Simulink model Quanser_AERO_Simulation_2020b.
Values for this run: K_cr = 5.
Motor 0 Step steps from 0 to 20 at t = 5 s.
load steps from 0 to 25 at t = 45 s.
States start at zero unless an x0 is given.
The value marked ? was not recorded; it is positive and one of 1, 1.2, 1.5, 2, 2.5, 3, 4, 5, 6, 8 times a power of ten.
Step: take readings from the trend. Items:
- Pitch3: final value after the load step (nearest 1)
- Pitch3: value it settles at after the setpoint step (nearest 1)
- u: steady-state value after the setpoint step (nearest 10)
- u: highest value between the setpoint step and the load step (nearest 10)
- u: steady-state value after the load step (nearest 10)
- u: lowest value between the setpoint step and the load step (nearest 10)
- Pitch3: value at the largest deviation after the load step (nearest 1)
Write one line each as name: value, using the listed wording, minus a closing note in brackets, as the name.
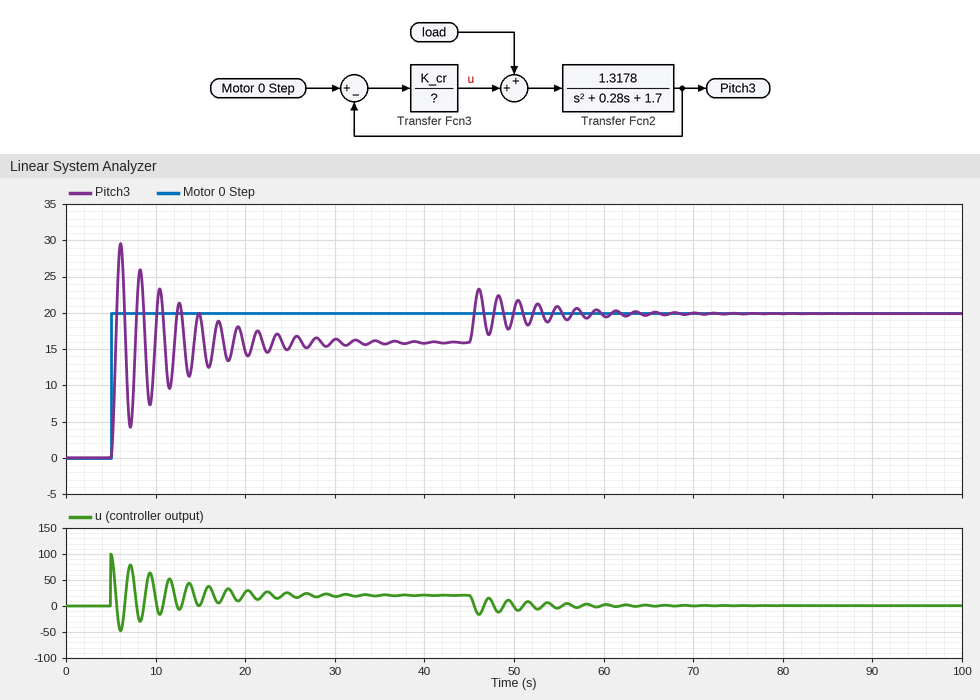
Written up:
Pitch3: final value after the load step: 20
Pitch3: value it settles at after the setpoint step: 16
u: steady-state value after the setpoint step: 20
u: highest value between the setpoint step and the load step: 100
u: steady-state value after the load step: 0
u: lowest value between the setpoint step and the load step: -50
Pitch3: value at the largest deviation after the load step: 23
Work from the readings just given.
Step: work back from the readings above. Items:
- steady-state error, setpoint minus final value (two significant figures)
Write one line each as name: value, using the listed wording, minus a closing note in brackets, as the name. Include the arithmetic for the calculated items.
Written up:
steady-state error, setpoint minus final value: 20 - 16 = 4.0
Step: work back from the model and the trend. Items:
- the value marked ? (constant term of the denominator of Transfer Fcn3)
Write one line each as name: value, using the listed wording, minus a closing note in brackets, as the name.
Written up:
the value marked ?: 1
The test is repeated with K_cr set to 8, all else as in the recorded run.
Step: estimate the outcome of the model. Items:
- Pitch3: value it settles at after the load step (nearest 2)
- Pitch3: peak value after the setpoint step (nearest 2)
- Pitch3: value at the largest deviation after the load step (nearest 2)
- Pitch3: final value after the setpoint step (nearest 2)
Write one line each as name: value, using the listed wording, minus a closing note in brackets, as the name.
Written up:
Pitch3: value it settles at after the load step: 20
Pitch3: peak value after the setpoint step: 32
Pitch3: value at the largest deviation after the load step: 22
Pitch3: final value after the setpoint step: 18
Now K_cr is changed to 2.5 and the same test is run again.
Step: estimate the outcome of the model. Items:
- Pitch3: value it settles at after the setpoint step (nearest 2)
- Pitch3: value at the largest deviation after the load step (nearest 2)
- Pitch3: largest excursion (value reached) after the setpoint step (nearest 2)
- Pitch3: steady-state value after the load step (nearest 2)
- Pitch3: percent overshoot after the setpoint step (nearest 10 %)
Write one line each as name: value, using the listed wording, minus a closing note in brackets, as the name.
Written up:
Pitch3: value it settles at after the setpoint step: 14
Pitch3: value at the largest deviation after the load step: 26
Pitch3: largest excursion (value reached) after the setpoint step: 24
Pitch3: steady-state value after the load step: 20
Pitch3: percent overshoot after the setpoint step: 80 %
